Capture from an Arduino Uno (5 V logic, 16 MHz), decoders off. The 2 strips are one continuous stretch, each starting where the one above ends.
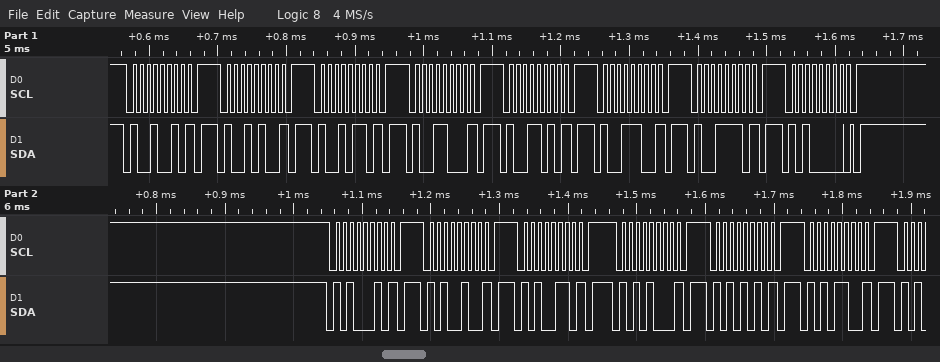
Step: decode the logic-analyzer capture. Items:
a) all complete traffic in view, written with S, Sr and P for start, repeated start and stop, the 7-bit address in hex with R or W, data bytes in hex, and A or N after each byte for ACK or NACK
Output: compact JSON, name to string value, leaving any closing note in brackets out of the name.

{"all complete traffic in view, written with S, Sr and P for start, repeated start and stop, the 7-bit address in hex with R or W, data bytes in hex, and A or N after each byte for ACK or NACK": "S 49W N P S 4AW N P S 4BW N P S 4CW N P S 4DW N P S 4EW N P S 4FW N P S 50W A P S 51W N P S 52W N P S 53W N P S 54W N P S 55W N P S 56W N P"}
